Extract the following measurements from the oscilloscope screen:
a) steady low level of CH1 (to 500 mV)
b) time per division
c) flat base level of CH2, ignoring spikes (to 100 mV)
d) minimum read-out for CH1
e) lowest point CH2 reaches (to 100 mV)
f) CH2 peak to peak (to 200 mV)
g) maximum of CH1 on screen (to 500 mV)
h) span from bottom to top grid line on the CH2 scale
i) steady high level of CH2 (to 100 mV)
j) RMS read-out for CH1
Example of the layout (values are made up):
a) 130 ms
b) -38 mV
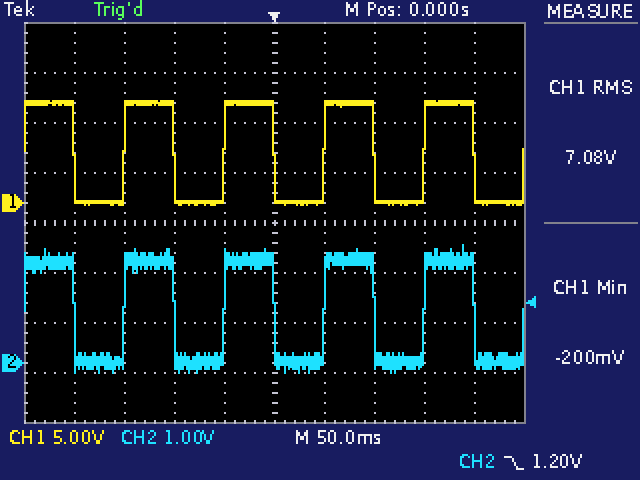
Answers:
a) 0.0 V
b) 50 ms
c) 0.0 V
d) -200 mV
e) -200 mV
f) 2.6 V
g) 10.0 V
h) 8 V
i) 2.0 V
j) 7.08 V
